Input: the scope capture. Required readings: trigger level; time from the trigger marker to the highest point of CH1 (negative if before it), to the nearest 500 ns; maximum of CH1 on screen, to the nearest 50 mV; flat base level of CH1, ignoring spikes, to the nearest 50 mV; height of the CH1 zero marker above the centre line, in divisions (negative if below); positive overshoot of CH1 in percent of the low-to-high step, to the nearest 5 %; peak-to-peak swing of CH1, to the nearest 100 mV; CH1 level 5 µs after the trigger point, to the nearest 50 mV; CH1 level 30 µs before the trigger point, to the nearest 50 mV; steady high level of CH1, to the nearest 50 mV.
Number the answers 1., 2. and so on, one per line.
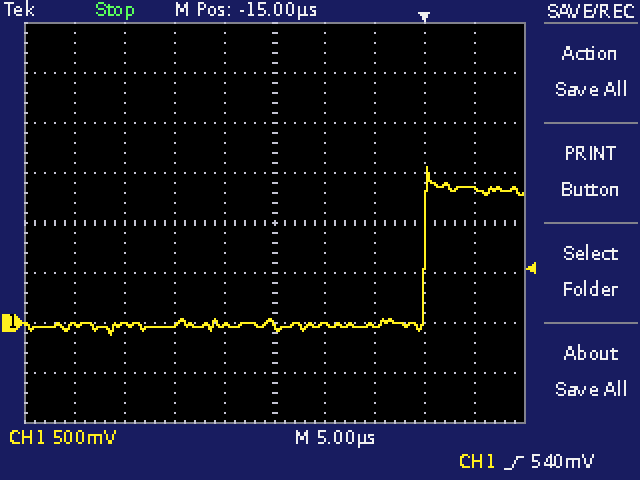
1. 540 mV
2. +500 ns
3. 1.55 V
4. -50 mV
5. -2.0 div
6. 15 %
7. 1.70 V
8. 1.35 V
9. 0 mV
10. 1.35 V
